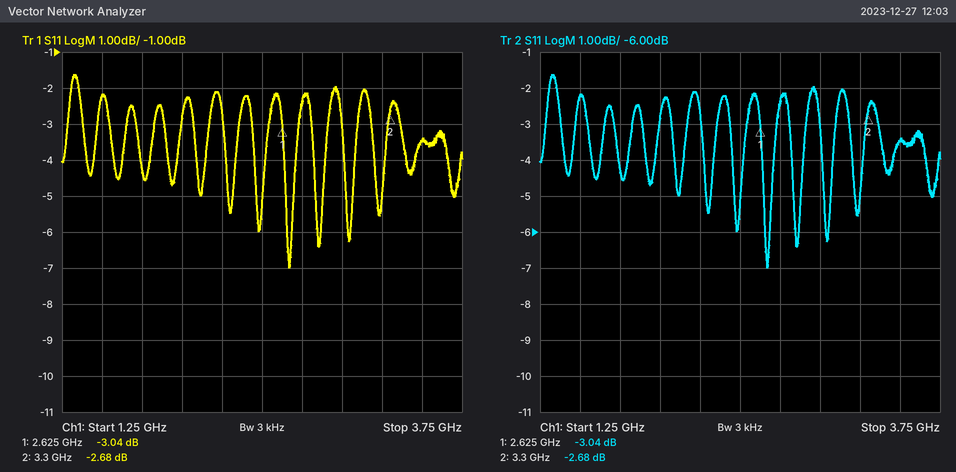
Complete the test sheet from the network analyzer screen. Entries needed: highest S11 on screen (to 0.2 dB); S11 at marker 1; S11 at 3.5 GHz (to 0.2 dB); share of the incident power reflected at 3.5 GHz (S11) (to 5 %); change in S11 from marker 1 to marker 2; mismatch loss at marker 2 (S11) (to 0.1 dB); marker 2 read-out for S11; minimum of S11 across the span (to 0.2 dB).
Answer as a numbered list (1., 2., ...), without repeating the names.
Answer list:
1. -1.6 dB
2. -3.04 dB
3. -3.4 dB
4. 45 %
5. 0.36 dB
6. 3.4 dB
7. -2.68 dB
8. -7.0 dB
